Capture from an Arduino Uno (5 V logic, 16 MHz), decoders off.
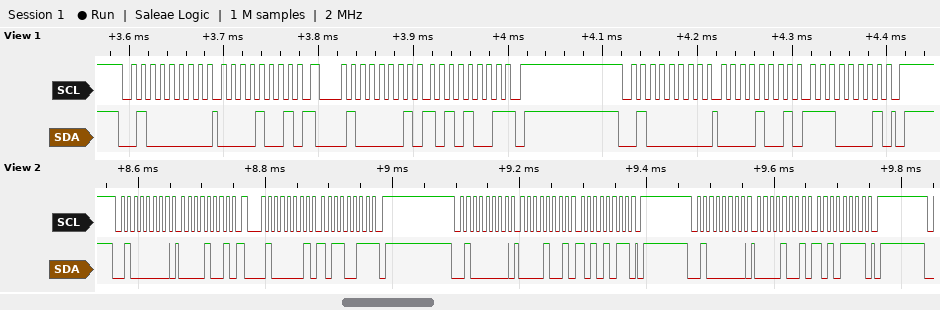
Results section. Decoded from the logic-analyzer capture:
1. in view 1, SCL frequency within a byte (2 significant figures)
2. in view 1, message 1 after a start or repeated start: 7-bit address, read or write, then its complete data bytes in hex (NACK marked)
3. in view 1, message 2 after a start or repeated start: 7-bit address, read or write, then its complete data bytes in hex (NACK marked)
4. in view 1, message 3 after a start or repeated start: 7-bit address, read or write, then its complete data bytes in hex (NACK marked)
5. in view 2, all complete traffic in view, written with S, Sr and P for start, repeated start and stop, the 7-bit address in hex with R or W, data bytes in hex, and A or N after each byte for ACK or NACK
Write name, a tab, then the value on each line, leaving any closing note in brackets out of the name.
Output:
in view 1, SCL frequency within a byte	100 kHz
in view 1, message 1 after a start or repeated start: 7-bit address, read or write, then its complete data bytes in hex	0x20 write: 09
in view 1, message 2 after a start or repeated start: 7-bit address, read or write, then its complete data bytes in hex	0x20 read: A9 NACK
in view 1, message 3 after a start or repeated start: 7-bit address, read or write, then its complete data bytes in hex	0x20 write: 09 E1
in view 2, all complete traffic in view, written with S, Sr and P for start, repeated start and stop, the 7-bit address in hex with R or W, data bytes in hex, and A or N after each byte for ACK or NACK	S 20W A 09 A Sr 20R A B3 N P S 20W A 09 A AB A P S 20W A 09 A AF A P
